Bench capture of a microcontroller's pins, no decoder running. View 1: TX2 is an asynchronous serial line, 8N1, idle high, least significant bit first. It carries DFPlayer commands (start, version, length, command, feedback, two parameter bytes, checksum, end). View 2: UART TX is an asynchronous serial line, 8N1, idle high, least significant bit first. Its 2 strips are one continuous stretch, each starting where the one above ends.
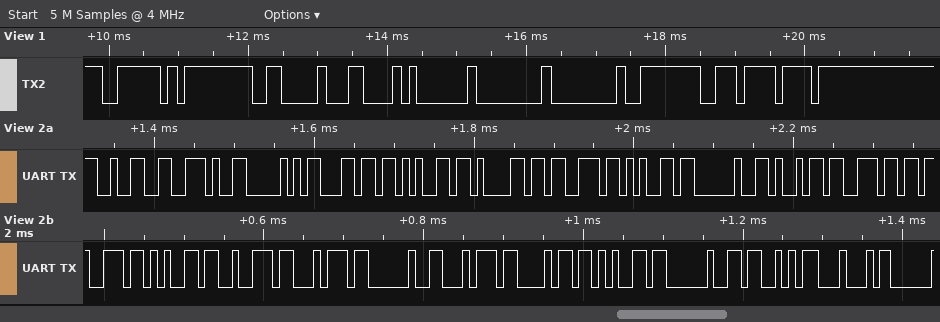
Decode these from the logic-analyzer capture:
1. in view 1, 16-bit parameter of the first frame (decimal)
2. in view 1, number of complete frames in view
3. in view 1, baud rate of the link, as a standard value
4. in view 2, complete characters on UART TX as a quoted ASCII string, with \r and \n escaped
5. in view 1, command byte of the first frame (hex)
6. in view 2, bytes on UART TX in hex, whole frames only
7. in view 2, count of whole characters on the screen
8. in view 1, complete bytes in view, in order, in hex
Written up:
0
10
9600 baud
"2.Please insert the SD"
0x0C
0x32 0x2E 0x50 0x6C 0x65 0x61 0x73 0x65 0x20 0x69 0x6E 0x73 0x65 0x72 0x74 0x20 0x74 0x68 0x65 0x20 0x53 0x44
22
7E FF 06 0C 01 00 00 FE EE EF
